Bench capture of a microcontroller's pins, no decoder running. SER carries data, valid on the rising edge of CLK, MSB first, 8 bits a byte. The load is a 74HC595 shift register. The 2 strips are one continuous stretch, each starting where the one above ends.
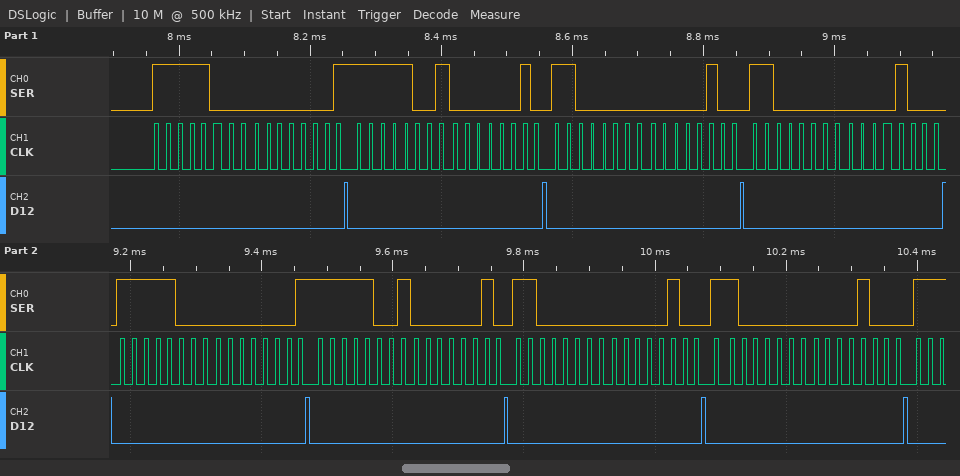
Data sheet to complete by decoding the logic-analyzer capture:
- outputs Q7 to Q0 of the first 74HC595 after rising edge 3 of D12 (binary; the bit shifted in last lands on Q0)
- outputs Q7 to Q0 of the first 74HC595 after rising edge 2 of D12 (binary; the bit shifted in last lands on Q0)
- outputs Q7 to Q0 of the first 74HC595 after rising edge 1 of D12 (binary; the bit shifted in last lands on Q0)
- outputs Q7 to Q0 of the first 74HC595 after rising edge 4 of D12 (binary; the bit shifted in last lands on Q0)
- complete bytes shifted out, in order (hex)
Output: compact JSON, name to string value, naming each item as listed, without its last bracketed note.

{"outputs Q7 to Q0 of the first 74HC595 after rising edge 3 of D12": "00000100", "outputs Q7 to Q0 of the first 74HC595 after rising edge 2 of D12": "00000010", "outputs Q7 to Q0 of the first 74HC595 after rising edge 1 of D12": "00000001", "outputs Q7 to Q0 of the first 74HC595 after rising edge 4 of D12": "00001000", "complete bytes shifted out, in order": "F8 01 F9 02 C0 04 C0 08 F8 01 F9 02 C0 04 C0 08"}
